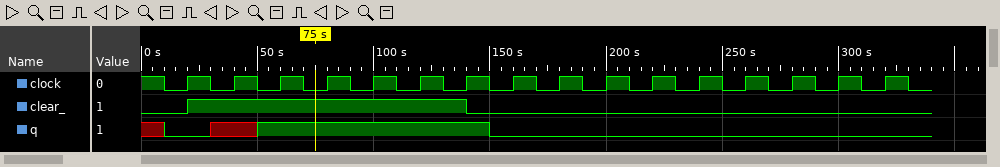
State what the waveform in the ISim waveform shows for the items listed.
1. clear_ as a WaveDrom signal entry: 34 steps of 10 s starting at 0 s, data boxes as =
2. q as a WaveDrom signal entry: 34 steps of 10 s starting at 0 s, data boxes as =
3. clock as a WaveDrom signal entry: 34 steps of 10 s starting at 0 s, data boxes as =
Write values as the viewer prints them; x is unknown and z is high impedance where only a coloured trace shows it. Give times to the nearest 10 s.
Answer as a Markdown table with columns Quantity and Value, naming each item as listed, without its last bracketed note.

| Quantity | Value |
|---|---|
| clear_ as a WaveDrom signal entry: 34 steps of 10 s starting at 0 s, data boxes as = | {name: 'clear_', wave: '0.1...........0...................'} |
| q as a WaveDrom signal entry: 34 steps of 10 s starting at 0 s, data boxes as = | {name: 'q', wave: 'x0.x.1.........0..................'} |
| clock as a WaveDrom signal entry: 34 steps of 10 s starting at 0 s, data boxes as = | {name: 'clock', wave: '1010101010101010101010101010101010'} |
